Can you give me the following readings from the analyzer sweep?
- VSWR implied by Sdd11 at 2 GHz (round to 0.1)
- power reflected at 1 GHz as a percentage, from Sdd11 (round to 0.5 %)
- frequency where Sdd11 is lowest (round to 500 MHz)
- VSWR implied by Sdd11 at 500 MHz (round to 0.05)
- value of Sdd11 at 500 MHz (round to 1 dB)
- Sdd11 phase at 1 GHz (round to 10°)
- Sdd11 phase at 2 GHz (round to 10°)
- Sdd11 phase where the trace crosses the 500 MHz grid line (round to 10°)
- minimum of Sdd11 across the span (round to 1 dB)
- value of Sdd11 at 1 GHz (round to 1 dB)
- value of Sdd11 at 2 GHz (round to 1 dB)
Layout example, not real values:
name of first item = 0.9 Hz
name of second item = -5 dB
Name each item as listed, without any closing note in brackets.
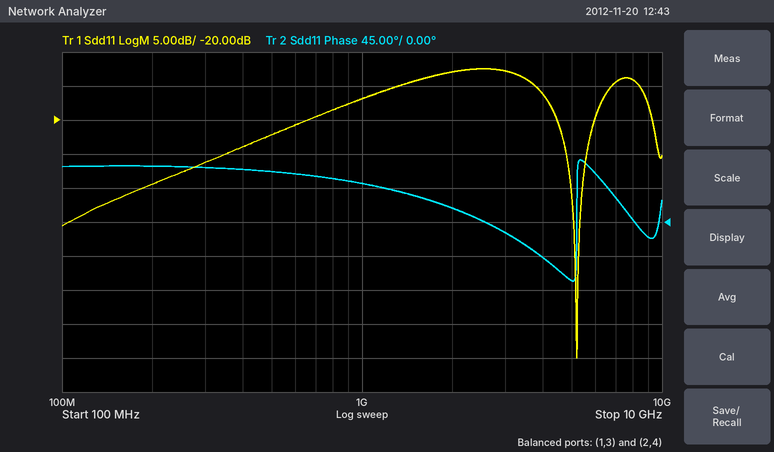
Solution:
VSWR implied by Sdd11 at 2 GHz = 1.6
power reflected at 1 GHz as a percentage, from Sdd11 = 2.0 %
frequency where Sdd11 is lowest = 5.0 GHz
VSWR implied by Sdd11 at 500 MHz = 1.15
value of Sdd11 at 500 MHz = -22 dB
Sdd11 phase at 1 GHz = 50°
Sdd11 phase at 2 GHz = 20°
Sdd11 phase where the trace crosses the 500 MHz grid line = 70°
minimum of Sdd11 across the span = -55 dB
value of Sdd11 at 1 GHz = -17 dB
value of Sdd11 at 2 GHz = -13 dB
